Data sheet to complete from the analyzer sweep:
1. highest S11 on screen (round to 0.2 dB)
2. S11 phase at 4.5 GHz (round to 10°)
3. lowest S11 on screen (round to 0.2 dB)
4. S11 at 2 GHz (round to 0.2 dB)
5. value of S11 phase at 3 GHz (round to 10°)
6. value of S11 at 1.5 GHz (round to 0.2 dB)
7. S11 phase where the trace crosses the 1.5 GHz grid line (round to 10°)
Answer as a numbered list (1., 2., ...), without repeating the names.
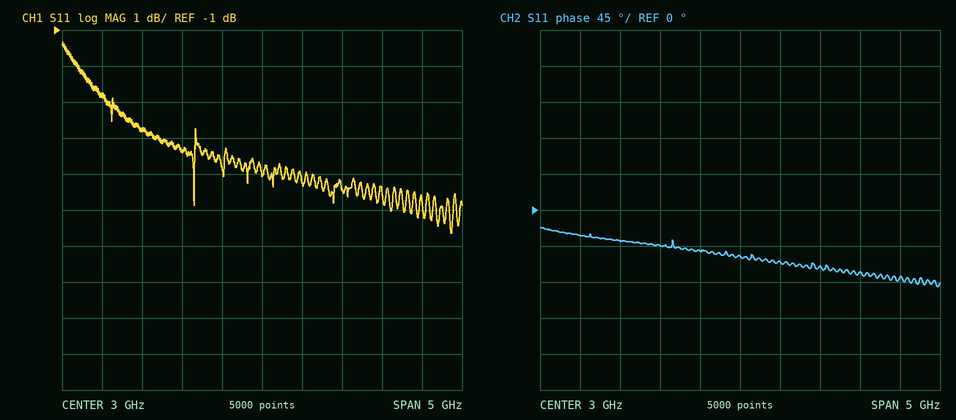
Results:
1. -1.4 dB
2. -80°
3. -6.6 dB
4. -4.4 dB
5. -60°
6. -3.8 dB
7. -40°
